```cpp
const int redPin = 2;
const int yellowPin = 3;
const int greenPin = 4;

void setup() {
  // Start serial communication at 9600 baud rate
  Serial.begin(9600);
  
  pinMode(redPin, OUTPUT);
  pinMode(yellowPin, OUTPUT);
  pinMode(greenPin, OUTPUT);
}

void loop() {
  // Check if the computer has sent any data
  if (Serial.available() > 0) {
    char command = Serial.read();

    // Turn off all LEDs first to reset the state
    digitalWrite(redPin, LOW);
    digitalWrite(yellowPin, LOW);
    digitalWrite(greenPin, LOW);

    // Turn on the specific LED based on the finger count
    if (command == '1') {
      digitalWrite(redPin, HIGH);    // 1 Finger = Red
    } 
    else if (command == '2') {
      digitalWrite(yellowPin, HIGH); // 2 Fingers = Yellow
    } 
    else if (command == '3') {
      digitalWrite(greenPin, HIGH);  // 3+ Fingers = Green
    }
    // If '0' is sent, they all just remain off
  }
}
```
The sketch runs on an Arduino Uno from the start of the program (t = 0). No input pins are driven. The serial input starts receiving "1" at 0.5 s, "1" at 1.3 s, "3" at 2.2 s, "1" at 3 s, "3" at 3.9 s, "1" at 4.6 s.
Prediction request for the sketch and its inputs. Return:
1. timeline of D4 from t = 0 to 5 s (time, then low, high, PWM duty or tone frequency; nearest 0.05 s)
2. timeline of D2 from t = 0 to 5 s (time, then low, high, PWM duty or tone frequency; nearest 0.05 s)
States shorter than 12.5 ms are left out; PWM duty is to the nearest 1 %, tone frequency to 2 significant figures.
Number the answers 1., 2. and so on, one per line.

1. 0 s low; 2.2 s high; 3 s low; 3.9 s high; 4.6 s low
2. 0 s low; 0.5 s high; 2.2 s low; 3 s high; 3.9 s low; 4.6 s high
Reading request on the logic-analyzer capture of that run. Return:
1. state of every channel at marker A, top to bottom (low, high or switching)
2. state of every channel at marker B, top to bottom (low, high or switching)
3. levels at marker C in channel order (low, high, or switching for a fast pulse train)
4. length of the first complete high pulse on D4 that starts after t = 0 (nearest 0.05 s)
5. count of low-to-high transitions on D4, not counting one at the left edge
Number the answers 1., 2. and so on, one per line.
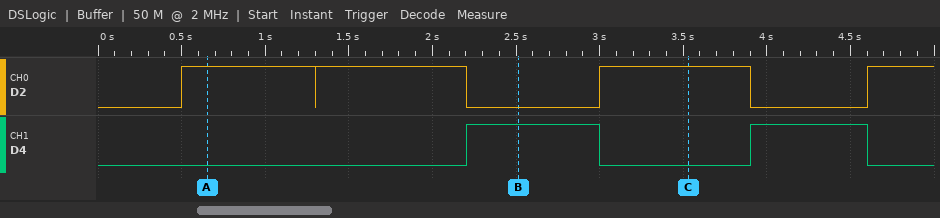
1. D2 high, D4 low
2. D2 low, D4 high
3. D2 high, D4 low
4. 0.80 s
5. 2
